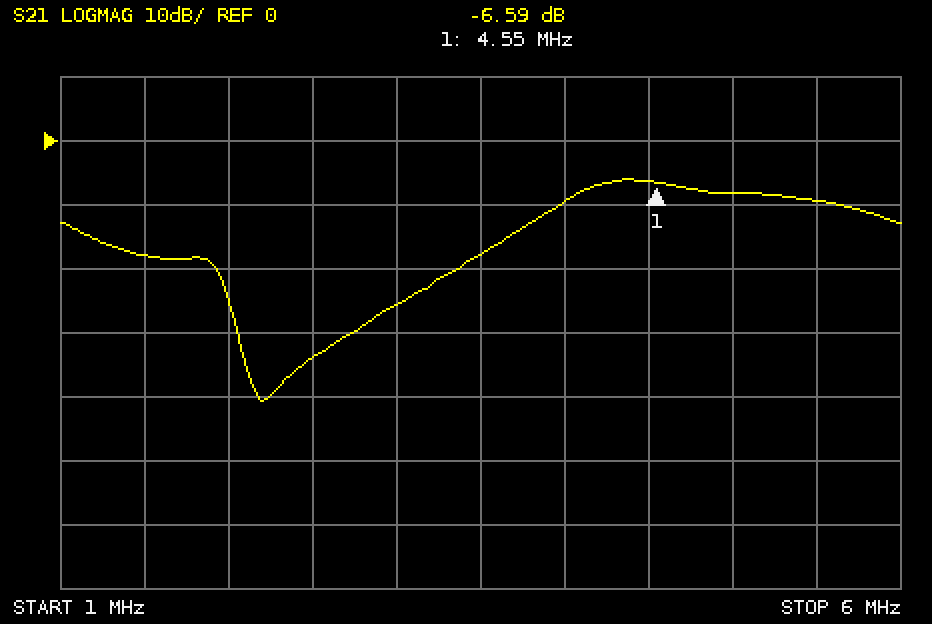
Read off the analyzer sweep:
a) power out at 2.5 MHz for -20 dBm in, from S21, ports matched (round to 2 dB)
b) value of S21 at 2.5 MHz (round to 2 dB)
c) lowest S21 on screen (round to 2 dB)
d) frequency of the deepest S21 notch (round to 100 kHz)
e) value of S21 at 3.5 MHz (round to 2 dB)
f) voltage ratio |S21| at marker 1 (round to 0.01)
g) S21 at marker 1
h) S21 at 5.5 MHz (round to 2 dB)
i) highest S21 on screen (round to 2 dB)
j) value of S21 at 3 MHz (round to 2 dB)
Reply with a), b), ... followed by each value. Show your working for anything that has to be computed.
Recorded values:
a) -20 dBm + (-34 dB) = -54 dBm
b) -34 dB
c) -40 dB
d) 2.2 MHz
e) -18 dB
f) 10^(-6.59/20) ≈ 0.47
g) -6.59 dB
h) -10 dB
i) -6 dB
j) -26 dB
